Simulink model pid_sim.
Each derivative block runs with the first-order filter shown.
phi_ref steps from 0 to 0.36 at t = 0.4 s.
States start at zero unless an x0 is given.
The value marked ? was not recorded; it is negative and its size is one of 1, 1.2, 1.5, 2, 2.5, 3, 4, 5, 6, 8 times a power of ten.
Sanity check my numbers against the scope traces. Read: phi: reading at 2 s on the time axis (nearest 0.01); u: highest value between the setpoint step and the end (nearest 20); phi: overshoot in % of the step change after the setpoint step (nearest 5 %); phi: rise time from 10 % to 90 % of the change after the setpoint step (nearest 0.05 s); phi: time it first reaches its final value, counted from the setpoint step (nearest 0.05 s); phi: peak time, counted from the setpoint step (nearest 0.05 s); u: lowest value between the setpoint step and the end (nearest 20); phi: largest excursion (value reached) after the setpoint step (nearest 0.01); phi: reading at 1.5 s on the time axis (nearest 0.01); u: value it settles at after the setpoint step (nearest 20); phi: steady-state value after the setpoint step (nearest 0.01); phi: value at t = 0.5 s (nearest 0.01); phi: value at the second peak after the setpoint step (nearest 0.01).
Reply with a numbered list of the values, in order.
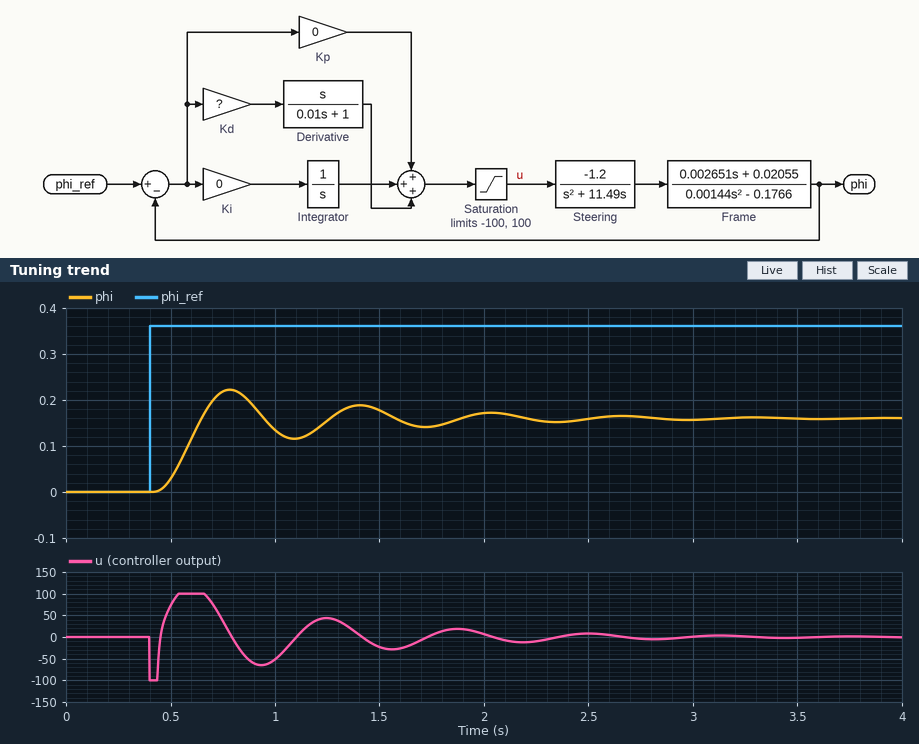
1. 0.17
2. 100
3. 40 %
4. 0.15 s
5. 0.25 s
6. 0.40 s
7. -100
8. 0.22
9. 0.18
10. 0
11. 0.16
12. 0.03
13. 0.19
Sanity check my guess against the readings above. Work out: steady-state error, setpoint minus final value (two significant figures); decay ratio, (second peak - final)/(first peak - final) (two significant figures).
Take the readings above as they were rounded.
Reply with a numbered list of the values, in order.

1. 0.20
2. 0.50
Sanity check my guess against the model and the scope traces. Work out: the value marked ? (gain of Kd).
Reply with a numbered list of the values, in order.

1. -120
